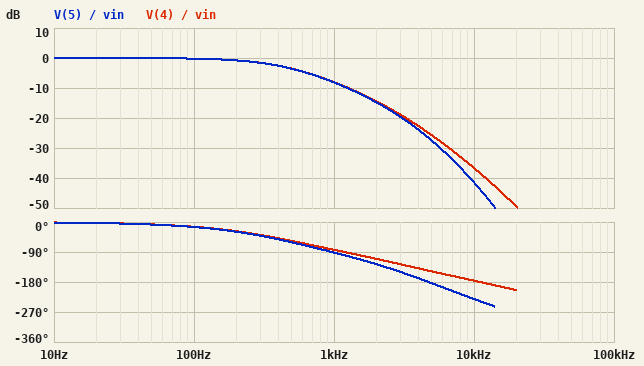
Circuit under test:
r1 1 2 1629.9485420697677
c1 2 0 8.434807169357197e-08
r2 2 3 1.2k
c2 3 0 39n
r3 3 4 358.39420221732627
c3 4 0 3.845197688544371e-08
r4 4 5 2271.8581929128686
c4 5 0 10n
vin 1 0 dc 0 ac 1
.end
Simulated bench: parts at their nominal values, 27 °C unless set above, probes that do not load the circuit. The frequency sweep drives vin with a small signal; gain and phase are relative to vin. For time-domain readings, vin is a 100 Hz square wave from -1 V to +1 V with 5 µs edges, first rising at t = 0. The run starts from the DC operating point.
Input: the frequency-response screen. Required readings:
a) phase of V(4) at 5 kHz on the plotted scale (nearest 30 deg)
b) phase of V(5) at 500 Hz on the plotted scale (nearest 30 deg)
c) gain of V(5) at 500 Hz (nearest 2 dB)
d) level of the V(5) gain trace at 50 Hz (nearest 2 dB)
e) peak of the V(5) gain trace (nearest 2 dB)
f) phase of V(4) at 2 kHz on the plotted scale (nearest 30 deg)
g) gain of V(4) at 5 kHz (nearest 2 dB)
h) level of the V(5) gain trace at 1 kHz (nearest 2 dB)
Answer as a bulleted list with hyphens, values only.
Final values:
- -150 deg
- -60 deg
- -4 dB
- 0 dB
- 0 dB
- -120 deg
- -26 dB
- -8 dB
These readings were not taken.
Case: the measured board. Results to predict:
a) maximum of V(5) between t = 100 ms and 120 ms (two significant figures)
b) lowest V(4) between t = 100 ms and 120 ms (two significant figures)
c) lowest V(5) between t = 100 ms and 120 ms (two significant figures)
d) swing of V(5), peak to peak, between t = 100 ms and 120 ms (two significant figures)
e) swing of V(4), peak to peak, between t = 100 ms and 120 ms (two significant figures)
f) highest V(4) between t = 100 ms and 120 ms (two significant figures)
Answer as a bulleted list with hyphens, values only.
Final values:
- 1.0 V
- -1.0 V
- -1.0 V
- 2.0 V
- 2.0 V
- 1.0 V
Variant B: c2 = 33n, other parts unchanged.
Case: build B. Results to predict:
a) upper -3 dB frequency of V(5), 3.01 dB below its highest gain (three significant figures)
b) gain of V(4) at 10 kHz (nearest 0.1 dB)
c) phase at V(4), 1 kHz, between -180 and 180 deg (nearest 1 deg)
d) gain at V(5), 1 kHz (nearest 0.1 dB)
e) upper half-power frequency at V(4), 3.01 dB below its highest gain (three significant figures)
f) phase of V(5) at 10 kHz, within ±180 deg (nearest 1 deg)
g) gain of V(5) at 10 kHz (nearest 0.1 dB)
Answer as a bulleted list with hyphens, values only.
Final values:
- 463 Hz
- -36.0 dB
- -82 deg
- -7.8 dB
- 465 Hz
- 132 deg
- -40.8 dB
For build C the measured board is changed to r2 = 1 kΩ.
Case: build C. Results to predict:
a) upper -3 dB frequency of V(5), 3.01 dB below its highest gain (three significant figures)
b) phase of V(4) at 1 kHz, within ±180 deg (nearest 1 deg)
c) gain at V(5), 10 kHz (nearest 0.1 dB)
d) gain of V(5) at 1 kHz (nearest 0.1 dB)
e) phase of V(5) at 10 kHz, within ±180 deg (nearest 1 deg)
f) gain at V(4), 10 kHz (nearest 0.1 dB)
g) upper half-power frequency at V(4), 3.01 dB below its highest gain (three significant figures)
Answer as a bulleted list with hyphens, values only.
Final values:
- 460 Hz
- -81 deg
- -40.2 dB
- -7.8 dB
- 132 deg
- -35.4 dB
- 462 Hz
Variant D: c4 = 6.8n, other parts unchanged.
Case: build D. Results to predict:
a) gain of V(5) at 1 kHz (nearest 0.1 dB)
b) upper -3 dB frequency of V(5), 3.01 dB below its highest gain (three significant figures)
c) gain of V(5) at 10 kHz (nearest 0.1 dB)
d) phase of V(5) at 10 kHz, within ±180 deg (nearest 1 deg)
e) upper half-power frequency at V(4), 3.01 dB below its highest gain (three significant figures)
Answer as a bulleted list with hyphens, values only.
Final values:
- -7.9 dB
- 457 Hz
- -39.5 dB
- 139 deg
- 458 Hz
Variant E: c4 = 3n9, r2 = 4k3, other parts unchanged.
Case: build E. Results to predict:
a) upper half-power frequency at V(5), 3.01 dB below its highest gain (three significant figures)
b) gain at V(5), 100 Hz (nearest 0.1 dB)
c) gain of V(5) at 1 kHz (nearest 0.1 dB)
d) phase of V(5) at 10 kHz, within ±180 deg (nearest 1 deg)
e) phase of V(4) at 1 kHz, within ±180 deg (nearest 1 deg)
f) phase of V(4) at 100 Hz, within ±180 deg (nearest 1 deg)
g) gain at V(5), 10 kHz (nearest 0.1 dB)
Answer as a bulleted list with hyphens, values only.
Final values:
- 288 Hz
- -0.5 dB
- -12.2 dB
- 140 deg
- -106 deg
- -22 deg
- -47.8 dB
